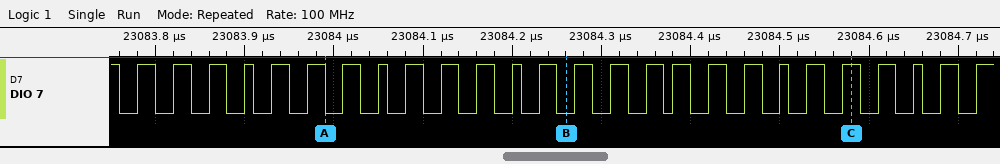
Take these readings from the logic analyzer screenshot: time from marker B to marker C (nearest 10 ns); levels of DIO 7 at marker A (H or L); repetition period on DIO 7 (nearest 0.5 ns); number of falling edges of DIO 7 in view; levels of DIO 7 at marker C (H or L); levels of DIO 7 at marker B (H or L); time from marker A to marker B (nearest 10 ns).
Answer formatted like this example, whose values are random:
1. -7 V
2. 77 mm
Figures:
1. 320 ns
2. DIO 7=L
3. 37.5 ns
4. 26
5. DIO 7=H
6. DIO 7=L
7. 270 ns
